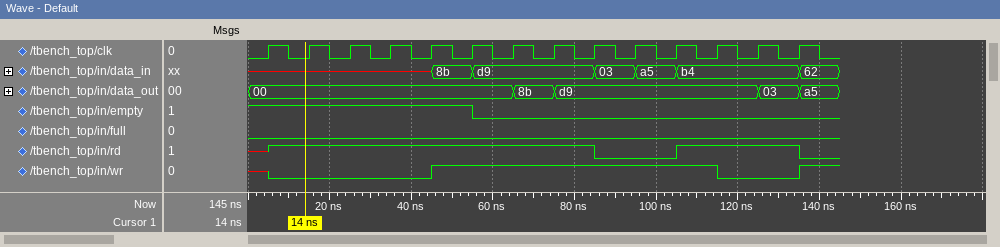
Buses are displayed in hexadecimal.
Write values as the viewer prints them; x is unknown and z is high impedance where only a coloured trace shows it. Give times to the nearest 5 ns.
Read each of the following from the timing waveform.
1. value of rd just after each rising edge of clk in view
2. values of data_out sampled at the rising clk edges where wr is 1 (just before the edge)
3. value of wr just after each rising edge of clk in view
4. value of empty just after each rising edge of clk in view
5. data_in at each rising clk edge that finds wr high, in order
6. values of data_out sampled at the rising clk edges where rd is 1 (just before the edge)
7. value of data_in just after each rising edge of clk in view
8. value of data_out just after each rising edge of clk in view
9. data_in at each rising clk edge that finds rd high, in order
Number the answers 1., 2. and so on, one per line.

1. 1 1 1 1 1 1 1 1 0 0 1 1 1 0
2. 00, 00, 8b, d9, d9, d9, d9
3. 0 0 0 0 1 1 1 1 1 1 1 0 0 1
4. 1 1 1 1 1 0 0 0 0 0 0 0 0 0
5. 8b, d9, d9, d9, 03, a5, b4
6. 00, 00, 00, 00, 00, 00, 8b, d9, d9, d9, 03
7. x, x, x, x, 8b, d9, d9, d9, 03, a5, b4, b4, b4, 62
8. 00, 00, 00, 00, 00, 00, 8b, d9, d9, d9, d9, d9, 03, a5
9. x, x, x, x, 8b, d9, d9, d9, b4, b4, b4
